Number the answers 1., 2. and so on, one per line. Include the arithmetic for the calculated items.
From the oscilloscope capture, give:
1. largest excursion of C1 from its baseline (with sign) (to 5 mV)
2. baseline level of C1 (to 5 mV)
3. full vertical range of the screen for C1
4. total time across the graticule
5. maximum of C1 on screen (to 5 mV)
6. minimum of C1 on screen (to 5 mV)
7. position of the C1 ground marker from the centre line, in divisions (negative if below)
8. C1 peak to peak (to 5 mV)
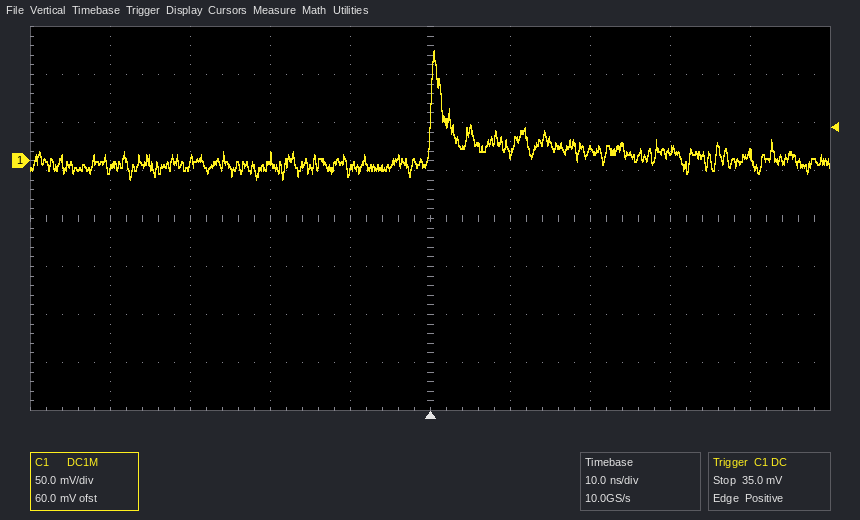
1. 115 mV − (0 mV) = +115 mV
2. 0 mV
3. 400 mV
4. 100 ns
5. 115 mV
6. -20 mV
7. +1.2 div
8. 115 mV − (-20 mV) = 135 mV
